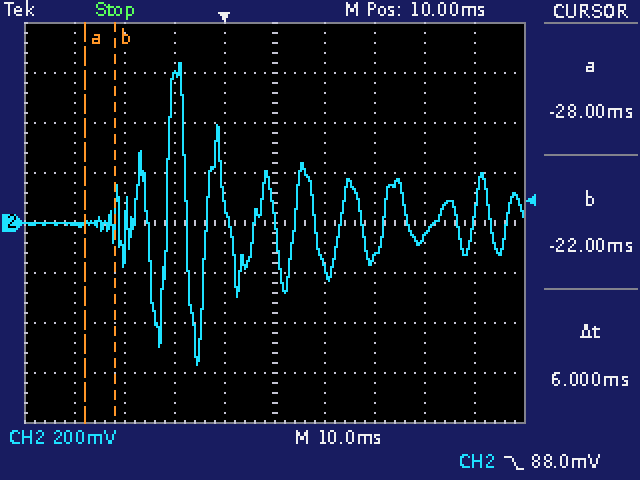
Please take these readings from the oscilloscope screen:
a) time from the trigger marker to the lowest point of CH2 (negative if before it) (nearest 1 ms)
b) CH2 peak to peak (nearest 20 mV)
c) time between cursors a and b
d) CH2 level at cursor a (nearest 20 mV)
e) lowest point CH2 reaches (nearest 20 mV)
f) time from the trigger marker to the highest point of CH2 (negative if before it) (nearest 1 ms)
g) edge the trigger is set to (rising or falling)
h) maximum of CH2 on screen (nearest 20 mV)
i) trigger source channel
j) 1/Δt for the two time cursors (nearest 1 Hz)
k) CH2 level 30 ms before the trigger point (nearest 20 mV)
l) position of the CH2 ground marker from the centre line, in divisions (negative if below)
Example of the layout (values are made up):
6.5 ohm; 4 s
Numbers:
-5 ms; 1.20 V; 6 ms; 0 mV; -560 mV; -9 ms; falling; 640 mV; CH2; 167 Hz; 0 mV; 0.0 div
